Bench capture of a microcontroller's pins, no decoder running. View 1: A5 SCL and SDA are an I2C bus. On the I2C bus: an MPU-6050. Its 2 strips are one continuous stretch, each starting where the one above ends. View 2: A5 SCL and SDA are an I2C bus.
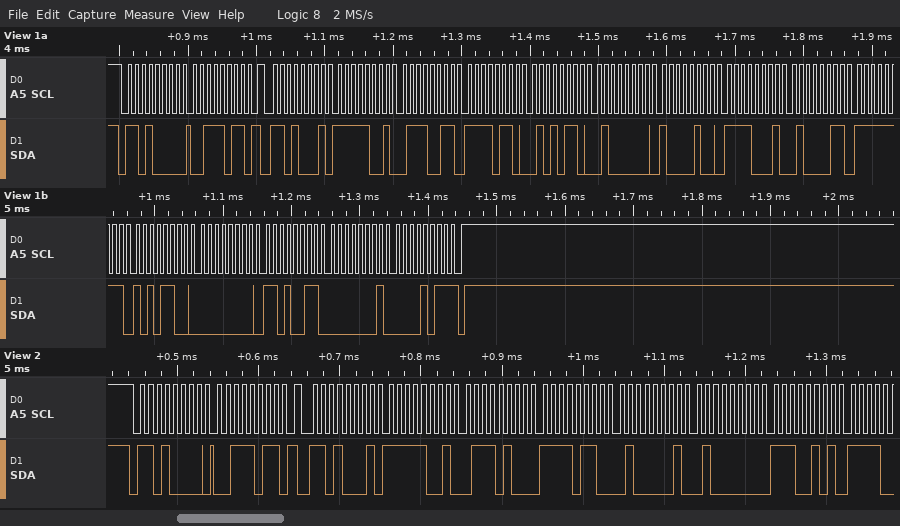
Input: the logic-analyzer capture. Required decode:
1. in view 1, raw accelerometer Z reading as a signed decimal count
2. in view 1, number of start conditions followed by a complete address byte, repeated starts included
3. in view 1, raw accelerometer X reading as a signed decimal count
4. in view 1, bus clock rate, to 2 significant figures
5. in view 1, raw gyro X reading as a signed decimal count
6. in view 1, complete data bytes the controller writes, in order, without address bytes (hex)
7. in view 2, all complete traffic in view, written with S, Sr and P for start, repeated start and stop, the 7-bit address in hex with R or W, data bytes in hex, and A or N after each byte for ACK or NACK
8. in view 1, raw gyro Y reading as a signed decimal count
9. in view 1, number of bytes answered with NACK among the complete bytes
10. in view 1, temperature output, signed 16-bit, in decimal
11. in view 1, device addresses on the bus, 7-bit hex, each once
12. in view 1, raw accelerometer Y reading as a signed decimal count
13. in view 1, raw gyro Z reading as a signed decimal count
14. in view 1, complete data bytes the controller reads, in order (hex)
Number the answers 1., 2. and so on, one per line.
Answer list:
1. 16516
2. 2
3. -1677
4. 100 kHz
5. -84
6. 3B
7. S 68W A 3B A Sr 68R A F9 A 74 A F6 A 41 A 40 A E5 A
8. 211
9. 1
10. -3773
11. 0x68
12. -2474
13. 267
14. F9 73 F6 56 40 84 F1 43 FF AC 00 D3 01 0B
